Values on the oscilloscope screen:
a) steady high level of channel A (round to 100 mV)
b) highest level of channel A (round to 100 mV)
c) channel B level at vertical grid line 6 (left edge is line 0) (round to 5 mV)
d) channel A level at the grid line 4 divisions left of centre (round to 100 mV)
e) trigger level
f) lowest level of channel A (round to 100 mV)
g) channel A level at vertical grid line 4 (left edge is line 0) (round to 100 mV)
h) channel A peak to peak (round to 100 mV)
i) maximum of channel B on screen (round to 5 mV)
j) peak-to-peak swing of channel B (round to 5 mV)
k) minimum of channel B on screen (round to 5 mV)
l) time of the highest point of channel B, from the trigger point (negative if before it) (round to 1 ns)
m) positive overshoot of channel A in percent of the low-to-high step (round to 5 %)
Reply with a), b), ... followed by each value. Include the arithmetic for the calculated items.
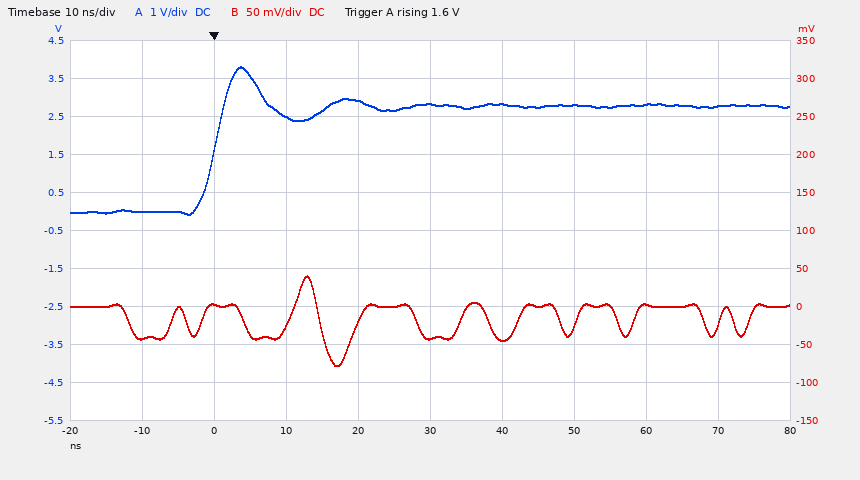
a) 2.8 V
b) 3.8 V
c) -45 mV
d) 0.0 V
e) 1.6 V
f) -100 mV
g) 2.9 V
h) 3.8 V − (-100 mV) = 3.9 V
i) 40 mV
j) 40 mV − (-80 mV) = 120 mV
k) -80 mV
l) +13 ns
m) 35 %
